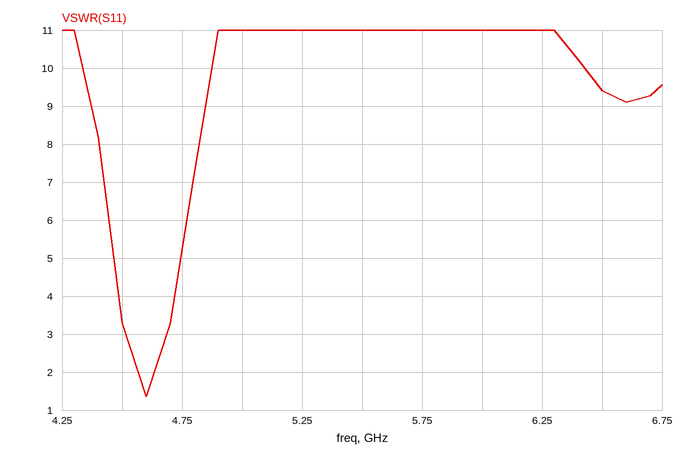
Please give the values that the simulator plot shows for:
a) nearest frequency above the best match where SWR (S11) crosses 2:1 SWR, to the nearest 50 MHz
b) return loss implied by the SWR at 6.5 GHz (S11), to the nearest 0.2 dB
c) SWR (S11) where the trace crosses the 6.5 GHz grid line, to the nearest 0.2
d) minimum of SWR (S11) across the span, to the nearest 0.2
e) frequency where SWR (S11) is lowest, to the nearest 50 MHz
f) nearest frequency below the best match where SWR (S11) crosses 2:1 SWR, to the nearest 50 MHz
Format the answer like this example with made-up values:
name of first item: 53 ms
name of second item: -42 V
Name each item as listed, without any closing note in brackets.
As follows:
nearest frequency above the best match where SWR (S11) crosses 2:1 SWR, to the nearest 50 MHz: 4.65 GHz
return loss implied by the SWR at 6.5 GHz (S11), to the nearest 0.2 dB: 1.8 dB
SWR (S11) where the trace crosses the 6.5 GHz grid line, to the nearest 0.2: 9.4
minimum of SWR (S11) across the span, to the nearest 0.2: 1.4
frequency where SWR (S11) is lowest, to the nearest 50 MHz: 4.60 GHz
nearest frequency below the best match where SWR (S11) crosses 2:1 SWR, to the nearest 50 MHz: 4.55 GHz
